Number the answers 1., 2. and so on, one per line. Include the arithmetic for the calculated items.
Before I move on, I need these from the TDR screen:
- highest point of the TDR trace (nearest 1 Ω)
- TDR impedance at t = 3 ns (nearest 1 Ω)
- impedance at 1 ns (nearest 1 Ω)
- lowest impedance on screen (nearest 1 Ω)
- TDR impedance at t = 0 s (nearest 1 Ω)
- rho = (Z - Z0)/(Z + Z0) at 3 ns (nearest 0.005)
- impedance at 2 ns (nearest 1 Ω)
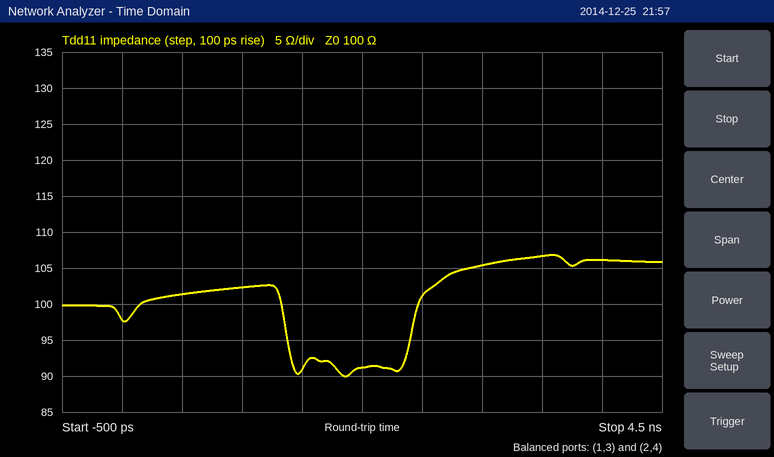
1. 107 Ω
2. 105 Ω
3. 102 Ω
4. 90 Ω
5. 98 Ω
6. (105 − 100)/(105 + 100) ≈ +0.0244, so +0.025 to the nearest 0.005
7. 91 Ω
